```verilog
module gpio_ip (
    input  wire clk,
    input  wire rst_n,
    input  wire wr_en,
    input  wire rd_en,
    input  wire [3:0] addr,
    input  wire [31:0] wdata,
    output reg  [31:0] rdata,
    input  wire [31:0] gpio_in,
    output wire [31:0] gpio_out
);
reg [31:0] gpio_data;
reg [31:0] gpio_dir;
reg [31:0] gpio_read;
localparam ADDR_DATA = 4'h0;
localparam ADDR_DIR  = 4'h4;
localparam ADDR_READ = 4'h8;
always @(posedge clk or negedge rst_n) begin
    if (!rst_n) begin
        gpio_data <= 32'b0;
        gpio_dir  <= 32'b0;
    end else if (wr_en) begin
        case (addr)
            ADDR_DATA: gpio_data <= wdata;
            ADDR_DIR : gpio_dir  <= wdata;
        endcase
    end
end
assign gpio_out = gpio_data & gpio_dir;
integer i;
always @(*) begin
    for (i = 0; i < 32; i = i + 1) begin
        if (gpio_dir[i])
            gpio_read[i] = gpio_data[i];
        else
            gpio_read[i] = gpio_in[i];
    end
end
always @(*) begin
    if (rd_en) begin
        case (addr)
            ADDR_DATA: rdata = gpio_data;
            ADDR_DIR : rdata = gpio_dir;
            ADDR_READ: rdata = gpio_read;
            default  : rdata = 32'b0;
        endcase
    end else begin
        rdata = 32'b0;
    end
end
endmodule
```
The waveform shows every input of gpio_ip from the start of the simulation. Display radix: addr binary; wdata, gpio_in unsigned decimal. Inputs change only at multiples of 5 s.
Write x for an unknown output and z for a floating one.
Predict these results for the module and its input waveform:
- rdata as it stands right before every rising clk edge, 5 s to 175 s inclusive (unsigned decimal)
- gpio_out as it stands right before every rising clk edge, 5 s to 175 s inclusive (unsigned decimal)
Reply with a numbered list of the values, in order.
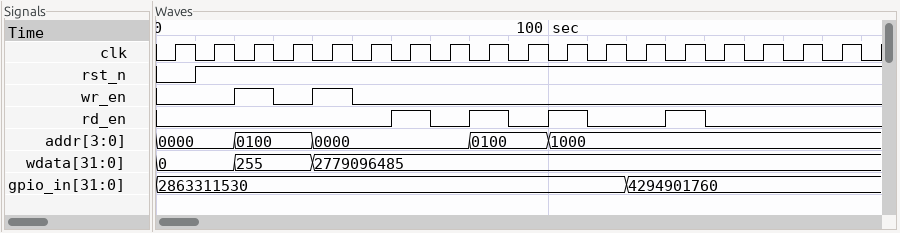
1. 0, 0, 0, 0, 0, 0, 2779096485, 0, 255, 0, 2863311525, 0, 0, 4294901925, 0, 0, 0, 0
2. 0, 0, 0, 0, 0, 165, 165, 165, 165, 165, 165, 165, 165, 165, 165, 165, 165, 165
